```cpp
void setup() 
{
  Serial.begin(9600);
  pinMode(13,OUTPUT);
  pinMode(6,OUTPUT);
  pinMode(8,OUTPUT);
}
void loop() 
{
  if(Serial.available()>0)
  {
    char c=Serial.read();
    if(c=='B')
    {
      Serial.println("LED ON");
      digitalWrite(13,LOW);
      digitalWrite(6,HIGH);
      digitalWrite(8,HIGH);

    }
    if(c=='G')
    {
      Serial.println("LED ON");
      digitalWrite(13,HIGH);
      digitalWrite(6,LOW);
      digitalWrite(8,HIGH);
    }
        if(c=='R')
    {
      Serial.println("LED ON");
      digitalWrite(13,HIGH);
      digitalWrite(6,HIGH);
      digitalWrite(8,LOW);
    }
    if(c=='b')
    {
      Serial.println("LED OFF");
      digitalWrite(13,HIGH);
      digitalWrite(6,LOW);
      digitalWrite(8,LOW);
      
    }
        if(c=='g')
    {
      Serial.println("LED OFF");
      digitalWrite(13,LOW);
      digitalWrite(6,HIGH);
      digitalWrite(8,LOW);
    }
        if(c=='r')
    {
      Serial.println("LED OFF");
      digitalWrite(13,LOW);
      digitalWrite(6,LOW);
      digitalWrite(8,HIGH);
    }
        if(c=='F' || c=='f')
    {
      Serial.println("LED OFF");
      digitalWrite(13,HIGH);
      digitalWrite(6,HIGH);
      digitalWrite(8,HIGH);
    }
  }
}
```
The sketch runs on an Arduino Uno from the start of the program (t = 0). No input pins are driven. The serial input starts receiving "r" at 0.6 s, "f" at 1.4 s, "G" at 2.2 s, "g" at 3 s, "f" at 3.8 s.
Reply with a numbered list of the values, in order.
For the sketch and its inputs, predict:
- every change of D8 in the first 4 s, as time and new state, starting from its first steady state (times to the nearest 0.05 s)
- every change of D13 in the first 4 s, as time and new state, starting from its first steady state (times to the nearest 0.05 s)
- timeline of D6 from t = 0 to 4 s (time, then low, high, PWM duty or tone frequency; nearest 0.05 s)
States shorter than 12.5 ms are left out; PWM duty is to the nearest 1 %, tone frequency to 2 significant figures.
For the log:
1. 0 s low; 0.6 s high; 3 s low; 3.8 s high
2. 0 s low; 1.4 s high; 3 s low; 3.8 s high
3. 0 s low; 1.4 s high; 2.2 s low; 3 s high
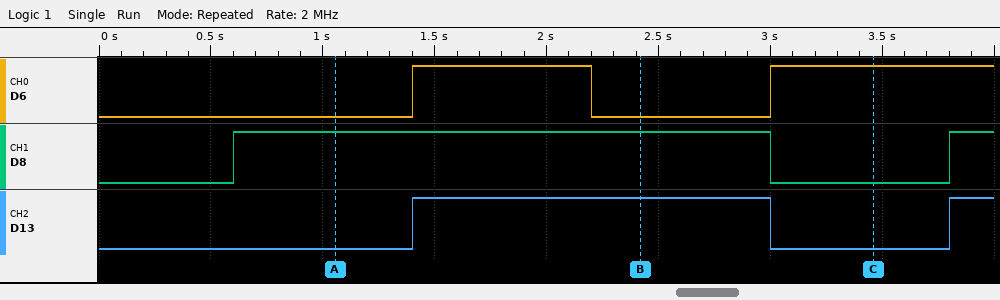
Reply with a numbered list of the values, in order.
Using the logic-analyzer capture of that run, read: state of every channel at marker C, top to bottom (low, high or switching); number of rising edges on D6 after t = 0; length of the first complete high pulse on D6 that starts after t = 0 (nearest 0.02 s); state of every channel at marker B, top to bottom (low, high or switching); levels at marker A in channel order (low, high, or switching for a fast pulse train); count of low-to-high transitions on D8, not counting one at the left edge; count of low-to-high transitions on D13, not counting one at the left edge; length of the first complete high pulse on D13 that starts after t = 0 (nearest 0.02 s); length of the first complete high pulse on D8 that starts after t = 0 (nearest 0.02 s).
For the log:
1. D6 high, D8 low, D13 low
2. 2
3. 0.80 s
4. D6 low, D8 high, D13 high
5. D6 low, D8 high, D13 low
6. 2
7. 2
8. 1.60 s
9. 2.40 s
